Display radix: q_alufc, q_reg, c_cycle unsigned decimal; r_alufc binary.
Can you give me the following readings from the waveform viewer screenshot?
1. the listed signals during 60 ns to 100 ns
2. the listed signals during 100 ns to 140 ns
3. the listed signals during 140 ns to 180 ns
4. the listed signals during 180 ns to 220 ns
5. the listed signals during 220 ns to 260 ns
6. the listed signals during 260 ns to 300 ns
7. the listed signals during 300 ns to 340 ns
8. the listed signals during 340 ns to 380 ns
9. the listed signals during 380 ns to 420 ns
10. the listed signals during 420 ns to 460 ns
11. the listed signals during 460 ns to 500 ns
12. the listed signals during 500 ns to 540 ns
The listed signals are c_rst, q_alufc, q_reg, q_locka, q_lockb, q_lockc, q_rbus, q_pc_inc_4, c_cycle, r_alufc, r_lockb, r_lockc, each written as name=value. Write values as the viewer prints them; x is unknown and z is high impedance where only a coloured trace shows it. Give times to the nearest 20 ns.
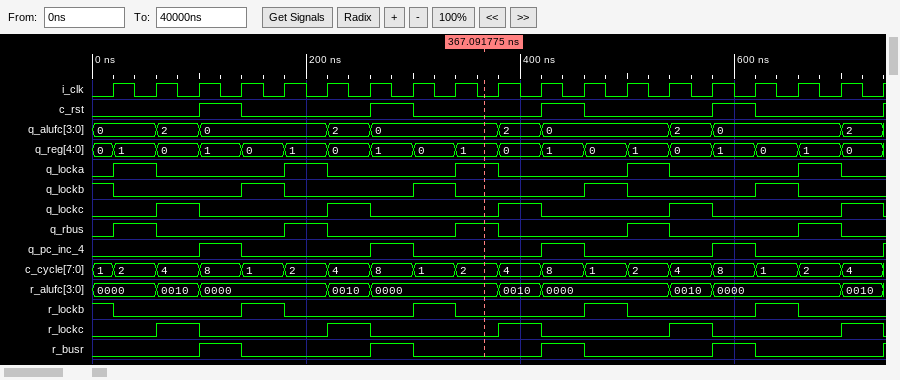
c_rst=0, q_alufc=2, q_reg=0, q_locka=0, q_lockb=0, q_lockc=1, q_rbus=0, q_pc_inc_4=0, c_cycle=4, r_alufc=0010, r_lockb=0, r_lockc=1
c_rst=1, q_alufc=0, q_reg=1, q_locka=0, q_lockb=0, q_lockc=0, q_rbus=0, q_pc_inc_4=1, c_cycle=8, r_alufc=0000, r_lockb=0, r_lockc=0
c_rst=0, q_alufc=0, q_reg=0, q_locka=0, q_lockb=1, q_lockc=0, q_rbus=0, q_pc_inc_4=0, c_cycle=1, r_alufc=0000, r_lockb=1, r_lockc=0
c_rst=0, q_alufc=0, q_reg=1, q_locka=1, q_lockb=0, q_lockc=0, q_rbus=1, q_pc_inc_4=0, c_cycle=2, r_alufc=0000, r_lockb=0, r_lockc=0
c_rst=0, q_alufc=2, q_reg=0, q_locka=0, q_lockb=0, q_lockc=1, q_rbus=0, q_pc_inc_4=0, c_cycle=4, r_alufc=0010, r_lockb=0, r_lockc=1
c_rst=1, q_alufc=0, q_reg=1, q_locka=0, q_lockb=0, q_lockc=0, q_rbus=0, q_pc_inc_4=1, c_cycle=8, r_alufc=0000, r_lockb=0, r_lockc=0
c_rst=0, q_alufc=0, q_reg=0, q_locka=0, q_lockb=1, q_lockc=0, q_rbus=0, q_pc_inc_4=0, c_cycle=1, r_alufc=0000, r_lockb=1, r_lockc=0
c_rst=0, q_alufc=0, q_reg=1, q_locka=1, q_lockb=0, q_lockc=0, q_rbus=1, q_pc_inc_4=0, c_cycle=2, r_alufc=0000, r_lockb=0, r_lockc=0
c_rst=0, q_alufc=2, q_reg=0, q_locka=0, q_lockb=0, q_lockc=1, q_rbus=0, q_pc_inc_4=0, c_cycle=4, r_alufc=0010, r_lockb=0, r_lockc=1
c_rst=1, q_alufc=0, q_reg=1, q_locka=0, q_lockb=0, q_lockc=0, q_rbus=0, q_pc_inc_4=1, c_cycle=8, r_alufc=0000, r_lockb=0, r_lockc=0
c_rst=0, q_alufc=0, q_reg=0, q_locka=0, q_lockb=1, q_lockc=0, q_rbus=0, q_pc_inc_4=0, c_cycle=1, r_alufc=0000, r_lockb=1, r_lockc=0
c_rst=0, q_alufc=0, q_reg=1, q_locka=1, q_lockb=0, q_lockc=0, q_rbus=1, q_pc_inc_4=0, c_cycle=2, r_alufc=0000, r_lockb=0, r_lockc=0
